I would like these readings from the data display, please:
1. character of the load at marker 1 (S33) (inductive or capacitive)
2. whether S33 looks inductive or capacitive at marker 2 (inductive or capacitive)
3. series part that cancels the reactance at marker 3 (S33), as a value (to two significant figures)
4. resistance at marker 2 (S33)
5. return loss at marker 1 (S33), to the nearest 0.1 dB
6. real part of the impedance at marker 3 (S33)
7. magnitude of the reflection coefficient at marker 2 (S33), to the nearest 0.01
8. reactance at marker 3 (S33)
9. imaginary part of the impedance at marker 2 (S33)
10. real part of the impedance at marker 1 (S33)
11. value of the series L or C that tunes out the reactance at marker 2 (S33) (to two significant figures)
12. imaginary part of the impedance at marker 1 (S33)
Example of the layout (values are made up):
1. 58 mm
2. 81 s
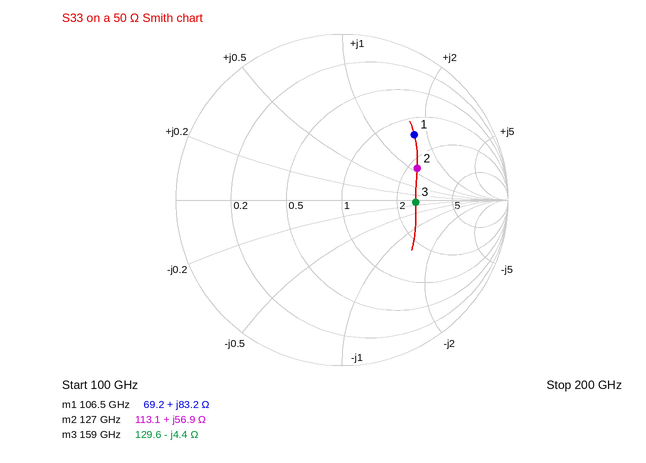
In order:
1. inductive
2. inductive
3. 4.4 pH
4. 113.1 Ω
5. 4.6 dB
6. 129.6 Ω
7. 0.49
8. -4.4 Ω
9. +56.9 Ω
10. 69.2 Ω
11. 22 fF
12. +83.2 Ω
